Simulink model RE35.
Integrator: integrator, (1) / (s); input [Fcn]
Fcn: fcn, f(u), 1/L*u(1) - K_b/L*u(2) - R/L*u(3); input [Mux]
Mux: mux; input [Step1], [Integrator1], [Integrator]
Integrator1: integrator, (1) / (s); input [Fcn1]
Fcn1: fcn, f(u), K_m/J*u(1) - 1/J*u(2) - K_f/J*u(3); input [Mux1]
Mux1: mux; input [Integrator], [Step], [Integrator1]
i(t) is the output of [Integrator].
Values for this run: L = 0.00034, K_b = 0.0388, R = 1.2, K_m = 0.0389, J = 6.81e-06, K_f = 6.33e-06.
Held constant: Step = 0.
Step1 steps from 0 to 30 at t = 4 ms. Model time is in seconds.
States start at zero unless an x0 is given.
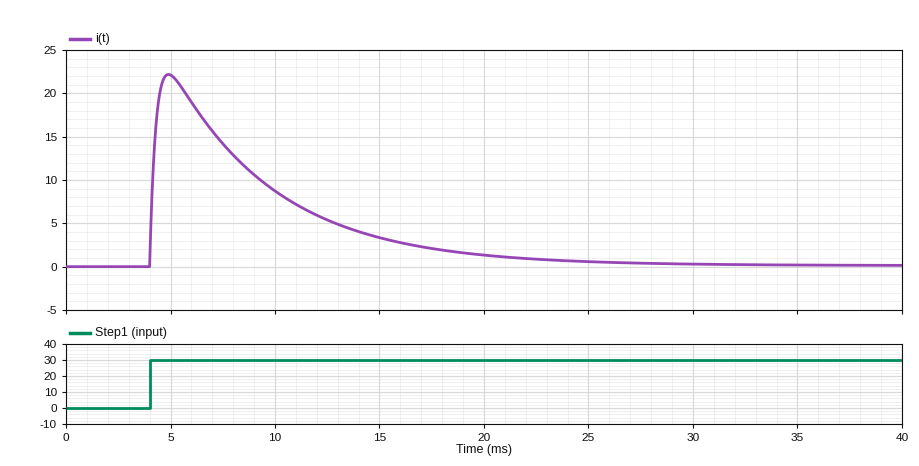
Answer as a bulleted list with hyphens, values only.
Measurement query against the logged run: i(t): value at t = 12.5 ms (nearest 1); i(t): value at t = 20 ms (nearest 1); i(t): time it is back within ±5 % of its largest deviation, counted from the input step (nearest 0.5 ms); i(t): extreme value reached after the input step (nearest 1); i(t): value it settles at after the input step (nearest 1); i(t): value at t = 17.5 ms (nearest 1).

- 5
- 1
- 16.5 ms
- 22
- 0
- 2
